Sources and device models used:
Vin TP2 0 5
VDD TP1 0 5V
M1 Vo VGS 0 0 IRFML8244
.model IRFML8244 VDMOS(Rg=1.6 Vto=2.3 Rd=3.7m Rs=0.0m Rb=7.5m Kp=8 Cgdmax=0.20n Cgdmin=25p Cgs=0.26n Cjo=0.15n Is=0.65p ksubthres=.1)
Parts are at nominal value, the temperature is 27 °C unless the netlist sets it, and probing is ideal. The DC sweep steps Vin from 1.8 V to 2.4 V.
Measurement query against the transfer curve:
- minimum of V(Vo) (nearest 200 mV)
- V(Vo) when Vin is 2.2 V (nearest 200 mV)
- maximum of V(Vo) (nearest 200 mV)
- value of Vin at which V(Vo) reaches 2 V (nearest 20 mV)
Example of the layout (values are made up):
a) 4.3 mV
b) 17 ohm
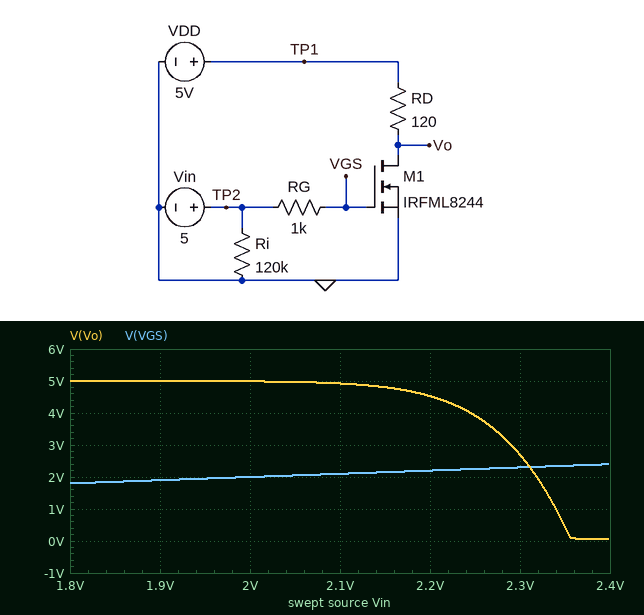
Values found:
a) 0 V
b) 4.6 V
c) 5.0 V
d) 2.32 V
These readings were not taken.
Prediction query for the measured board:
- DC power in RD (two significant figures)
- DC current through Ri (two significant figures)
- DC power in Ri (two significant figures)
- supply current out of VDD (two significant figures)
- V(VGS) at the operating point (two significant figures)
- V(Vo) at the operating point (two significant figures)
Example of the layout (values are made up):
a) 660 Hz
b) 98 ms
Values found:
a) 210 mW
b) 42 µA
c) 210 µW
d) 42 mA
e) 5.0 V
f) 2.1 mV
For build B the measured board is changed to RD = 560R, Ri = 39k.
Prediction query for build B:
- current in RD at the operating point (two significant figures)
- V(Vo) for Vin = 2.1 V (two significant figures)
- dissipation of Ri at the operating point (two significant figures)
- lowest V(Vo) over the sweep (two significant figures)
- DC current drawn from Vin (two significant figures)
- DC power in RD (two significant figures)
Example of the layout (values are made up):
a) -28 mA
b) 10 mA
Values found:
a) 8.9 mA
b) 4.6 V
c) 640 µW
d) 8.8 mV
e) 130 µA
f) 45 mW
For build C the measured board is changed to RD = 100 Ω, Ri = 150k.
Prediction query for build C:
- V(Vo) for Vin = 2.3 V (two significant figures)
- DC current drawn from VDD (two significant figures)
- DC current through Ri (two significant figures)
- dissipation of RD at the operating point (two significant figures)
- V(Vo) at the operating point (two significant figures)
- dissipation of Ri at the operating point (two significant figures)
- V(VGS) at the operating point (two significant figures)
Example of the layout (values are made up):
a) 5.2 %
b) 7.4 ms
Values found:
a) 3.1 V
b) 50 mA
c) 33 µA
d) 250 mW
e) 2.5 mV
f) 170 µW
g) 5.0 V
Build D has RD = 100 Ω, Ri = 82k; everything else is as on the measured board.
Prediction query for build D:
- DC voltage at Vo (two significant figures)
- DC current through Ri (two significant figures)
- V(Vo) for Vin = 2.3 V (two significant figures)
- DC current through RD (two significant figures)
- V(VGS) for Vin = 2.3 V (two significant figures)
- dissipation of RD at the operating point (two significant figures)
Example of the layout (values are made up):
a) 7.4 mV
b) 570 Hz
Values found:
a) 2.5 mV
b) 61 µA
c) 3.1 V
d) 50 mA
e) 2.3 V
f) 250 mW
